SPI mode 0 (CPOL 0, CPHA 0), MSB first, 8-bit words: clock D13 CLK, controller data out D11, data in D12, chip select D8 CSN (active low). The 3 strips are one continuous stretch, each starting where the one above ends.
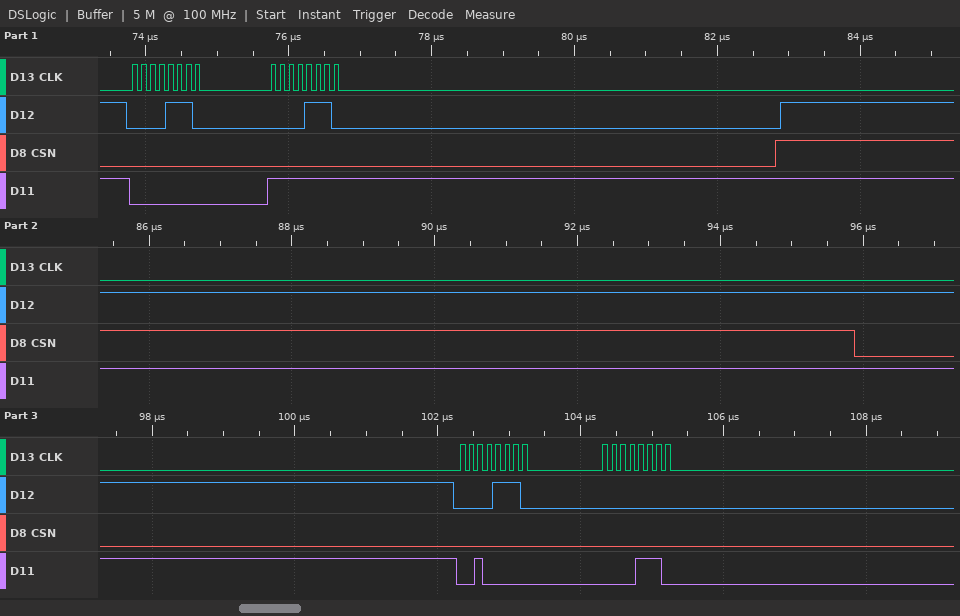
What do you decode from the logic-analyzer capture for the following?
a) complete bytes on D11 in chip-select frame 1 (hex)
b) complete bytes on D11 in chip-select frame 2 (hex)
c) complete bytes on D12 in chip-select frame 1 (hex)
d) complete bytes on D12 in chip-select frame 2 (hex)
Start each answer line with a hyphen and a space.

- 0x00 0xFF
- 0x20 0x0E
- 0x0E 0x0E
- 0x0E 0x00
